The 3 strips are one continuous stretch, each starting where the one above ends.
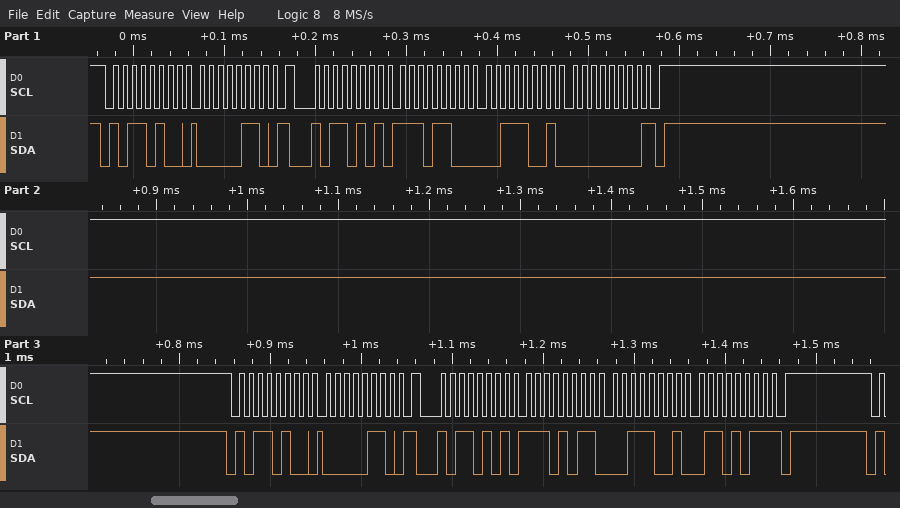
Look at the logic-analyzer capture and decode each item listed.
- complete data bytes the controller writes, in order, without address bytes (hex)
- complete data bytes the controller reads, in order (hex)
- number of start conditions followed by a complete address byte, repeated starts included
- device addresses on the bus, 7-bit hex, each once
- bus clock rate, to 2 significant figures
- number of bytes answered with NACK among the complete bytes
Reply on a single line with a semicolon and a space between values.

06 06; EC 39 00 EB 39 6B; 4; 0x5A; 100 kHz; 2
